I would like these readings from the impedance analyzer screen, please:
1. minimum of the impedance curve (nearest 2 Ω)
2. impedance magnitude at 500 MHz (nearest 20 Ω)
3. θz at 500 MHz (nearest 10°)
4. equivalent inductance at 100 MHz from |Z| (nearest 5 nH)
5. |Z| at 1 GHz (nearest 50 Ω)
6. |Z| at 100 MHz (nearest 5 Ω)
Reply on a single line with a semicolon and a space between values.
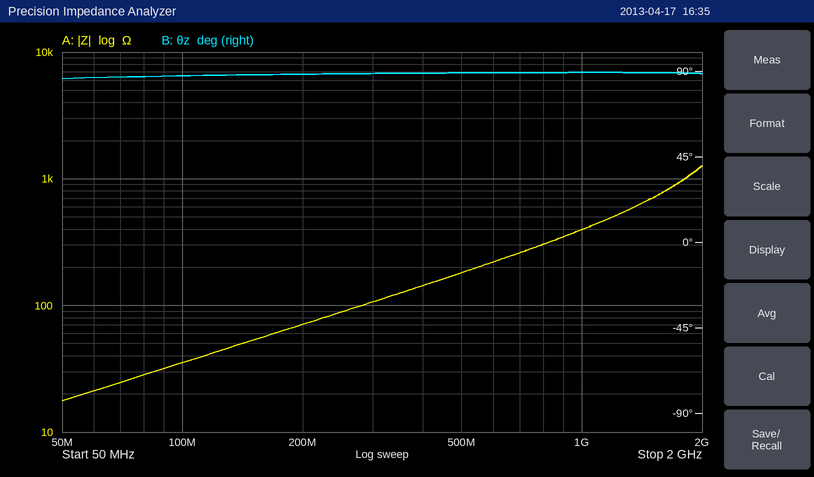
18 Ω; 180 Ω; 90°; 55 nH; 400 Ω; 35 Ω
